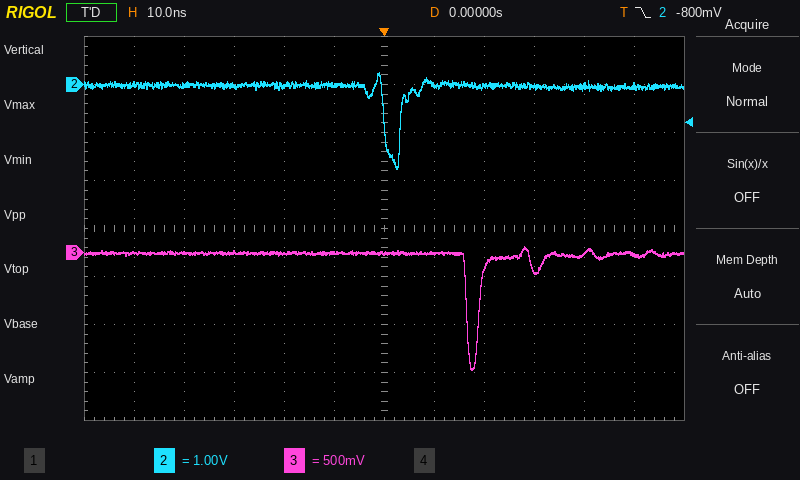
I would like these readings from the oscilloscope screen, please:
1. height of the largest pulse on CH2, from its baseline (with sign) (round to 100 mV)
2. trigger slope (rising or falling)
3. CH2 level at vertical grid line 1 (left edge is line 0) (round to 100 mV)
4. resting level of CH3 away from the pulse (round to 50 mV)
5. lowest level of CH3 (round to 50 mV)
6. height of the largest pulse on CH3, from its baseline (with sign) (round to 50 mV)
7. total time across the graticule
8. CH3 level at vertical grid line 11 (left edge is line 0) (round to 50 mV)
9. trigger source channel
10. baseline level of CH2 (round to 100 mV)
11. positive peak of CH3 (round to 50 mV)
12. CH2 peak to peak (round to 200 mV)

-1.7 V
falling
0.0 V
0 mV
-1.20 V
-1.20 V
120 ns
0 mV
CH2
0.0 V
50 mV
2.0 V
